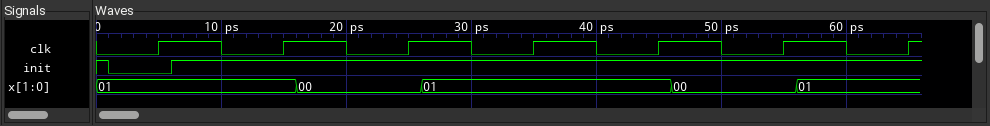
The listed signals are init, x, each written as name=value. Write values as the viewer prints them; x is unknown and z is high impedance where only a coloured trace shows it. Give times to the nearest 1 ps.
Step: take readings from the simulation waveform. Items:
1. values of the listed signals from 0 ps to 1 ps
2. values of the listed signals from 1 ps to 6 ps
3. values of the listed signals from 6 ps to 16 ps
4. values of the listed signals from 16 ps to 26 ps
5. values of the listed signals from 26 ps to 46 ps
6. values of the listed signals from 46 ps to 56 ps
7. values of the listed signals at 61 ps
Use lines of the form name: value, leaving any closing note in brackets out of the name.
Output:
values of the listed signals from 0 ps to 1 ps: init=1, x=01
values of the listed signals from 1 ps to 6 ps: init=0, x=01
values of the listed signals from 6 ps to 16 ps: init=1, x=01
values of the listed signals from 16 ps to 26 ps: init=1, x=00
values of the listed signals from 26 ps to 46 ps: init=1, x=01
values of the listed signals from 46 ps to 56 ps: init=1, x=00
values of the listed signals at 61 ps: init=1, x=01
